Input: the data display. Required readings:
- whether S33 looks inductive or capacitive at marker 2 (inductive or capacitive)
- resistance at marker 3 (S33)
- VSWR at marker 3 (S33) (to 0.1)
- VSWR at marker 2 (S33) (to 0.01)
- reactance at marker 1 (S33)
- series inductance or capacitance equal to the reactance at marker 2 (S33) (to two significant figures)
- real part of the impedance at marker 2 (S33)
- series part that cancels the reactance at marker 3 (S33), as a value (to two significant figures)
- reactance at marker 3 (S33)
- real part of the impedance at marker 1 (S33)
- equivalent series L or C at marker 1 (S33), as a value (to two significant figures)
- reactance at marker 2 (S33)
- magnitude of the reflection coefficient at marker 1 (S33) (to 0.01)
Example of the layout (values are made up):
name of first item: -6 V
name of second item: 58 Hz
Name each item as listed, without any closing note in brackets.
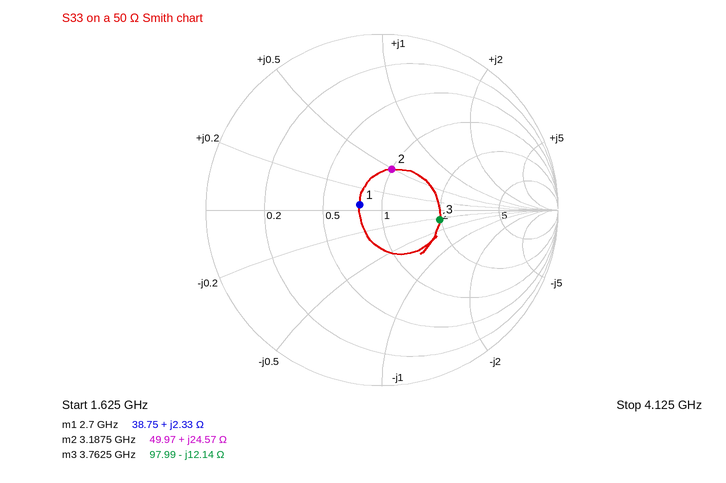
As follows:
whether S33 looks inductive or capacitive at marker 2: inductive
resistance at marker 3: 97.99 Ω
VSWR at marker 3 (S33): 2.0
VSWR at marker 2 (S33): 1.63
reactance at marker 1: +2.33 Ω
series inductance or capacitance equal to the reactance at marker 2 (S33): 1.2 nH
real part of the impedance at marker 2: 49.97 Ω
series part that cancels the reactance at marker 3 (S33), as a value: 510 pH
reactance at marker 3: -12.14 Ω
real part of the impedance at marker 1: 38.75 Ω
equivalent series L or C at marker 1 (S33), as a value: 140 pH
reactance at marker 2: +24.57 Ω
magnitude of the reflection coefficient at marker 1 (S33): 0.13
